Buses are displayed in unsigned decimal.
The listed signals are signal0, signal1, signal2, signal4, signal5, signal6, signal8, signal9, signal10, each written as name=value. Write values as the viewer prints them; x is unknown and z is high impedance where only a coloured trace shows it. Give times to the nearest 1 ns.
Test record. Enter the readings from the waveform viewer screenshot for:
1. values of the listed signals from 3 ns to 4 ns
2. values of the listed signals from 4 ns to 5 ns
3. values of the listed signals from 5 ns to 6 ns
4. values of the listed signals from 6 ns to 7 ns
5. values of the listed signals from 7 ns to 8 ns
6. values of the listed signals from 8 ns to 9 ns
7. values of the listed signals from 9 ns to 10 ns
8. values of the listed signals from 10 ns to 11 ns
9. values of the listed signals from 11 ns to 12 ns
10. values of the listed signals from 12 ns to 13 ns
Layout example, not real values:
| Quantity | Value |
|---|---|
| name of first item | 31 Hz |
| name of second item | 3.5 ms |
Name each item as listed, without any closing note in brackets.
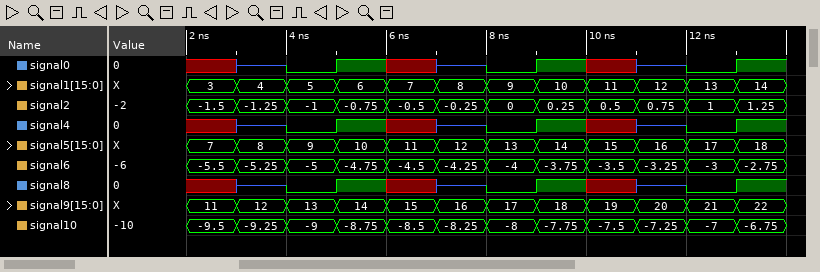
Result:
| Quantity | Value |
|---|---|
| values of the listed signals from 3 ns to 4 ns | signal0=z, signal1=4, signal2=-1.25, signal4=z, signal5=8, signal6=-5.25, signal8=z, signal9=12, signal10=-9.25 |
| values of the listed signals from 4 ns to 5 ns | signal0=0, signal1=5, signal2=-1, signal4=0, signal5=9, signal6=-5, signal8=0, signal9=13, signal10=-9 |
| values of the listed signals from 5 ns to 6 ns | signal0=1, signal1=6, signal2=-0.75, signal4=1, signal5=10, signal6=-4.75, signal8=1, signal9=14, signal10=-8.75 |
| values of the listed signals from 6 ns to 7 ns | signal0=x, signal1=7, signal2=-0.5, signal4=x, signal5=11, signal6=-4.5, signal8=x, signal9=15, signal10=-8.5 |
| values of the listed signals from 7 ns to 8 ns | signal0=z, signal1=8, signal2=-0.25, signal4=z, signal5=12, signal6=-4.25, signal8=z, signal9=16, signal10=-8.25 |
| values of the listed signals from 8 ns to 9 ns | signal0=0, signal1=9, signal2=0, signal4=0, signal5=13, signal6=-4, signal8=0, signal9=17, signal10=-8 |
| values of the listed signals from 9 ns to 10 ns | signal0=1, signal1=10, signal2=0.25, signal4=1, signal5=14, signal6=-3.75, signal8=1, signal9=18, signal10=-7.75 |
| values of the listed signals from 10 ns to 11 ns | signal0=x, signal1=11, signal2=0.5, signal4=x, signal5=15, signal6=-3.5, signal8=x, signal9=19, signal10=-7.5 |
| values of the listed signals from 11 ns to 12 ns | signal0=z, signal1=12, signal2=0.75, signal4=z, signal5=16, signal6=-3.25, signal8=z, signal9=20, signal10=-7.25 |
| values of the listed signals from 12 ns to 13 ns | signal0=0, signal1=13, signal2=1, signal4=0, signal5=17, signal6=-3, signal8=0, signal9=21, signal10=-7 |
